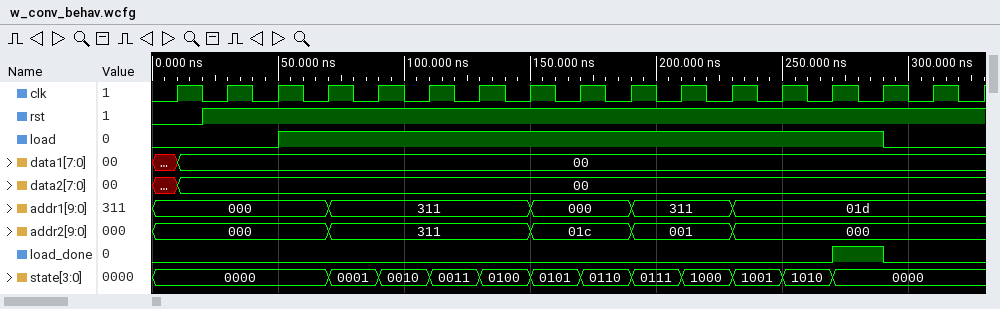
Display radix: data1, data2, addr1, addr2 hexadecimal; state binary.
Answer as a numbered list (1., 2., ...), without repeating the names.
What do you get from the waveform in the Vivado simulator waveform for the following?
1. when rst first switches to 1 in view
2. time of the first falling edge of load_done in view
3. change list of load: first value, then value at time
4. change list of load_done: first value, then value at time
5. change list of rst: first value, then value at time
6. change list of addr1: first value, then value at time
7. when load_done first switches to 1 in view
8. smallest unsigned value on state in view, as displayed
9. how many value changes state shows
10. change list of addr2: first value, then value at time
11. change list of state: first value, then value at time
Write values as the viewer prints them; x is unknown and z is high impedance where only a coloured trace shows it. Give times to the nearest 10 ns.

1. 20 ns
2. 290 ns
3. 0, 1 at 50 ns, 0 at 290 ns
4. 0, 1 at 270 ns, 0 at 290 ns
5. 0, 1 at 20 ns
6. 000, 311 at 70 ns, 000 at 150 ns, 311 at 190 ns, 01d at 230 ns
7. 270 ns
8. 0000
9. 11
10. 000, 311 at 70 ns, 01c at 150 ns, 001 at 190 ns, 000 at 230 ns
11. 0000, 0001 at 70 ns, 0010 at 90 ns, 0011 at 110 ns, 0100 at 130 ns, 0101 at 150 ns, 0110 at 170 ns, 0111 at 190 ns, 1000 at 210 ns, 1001 at 230 ns, 1010 at 250 ns, 0000 at 270 ns
